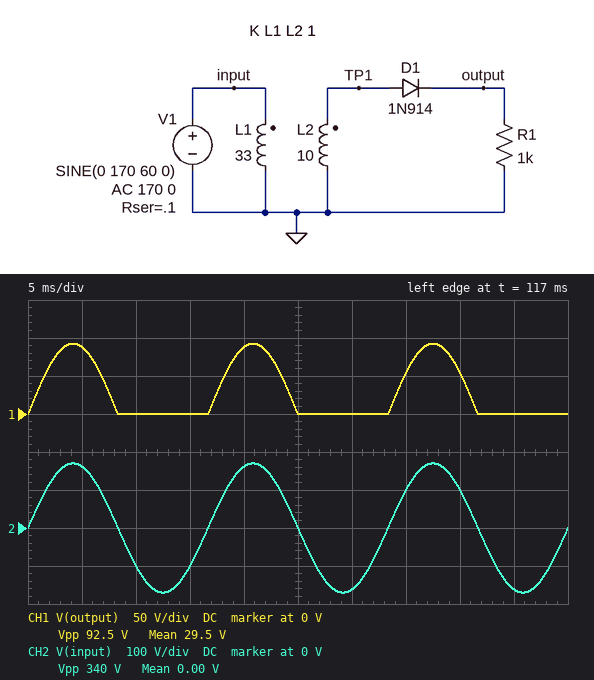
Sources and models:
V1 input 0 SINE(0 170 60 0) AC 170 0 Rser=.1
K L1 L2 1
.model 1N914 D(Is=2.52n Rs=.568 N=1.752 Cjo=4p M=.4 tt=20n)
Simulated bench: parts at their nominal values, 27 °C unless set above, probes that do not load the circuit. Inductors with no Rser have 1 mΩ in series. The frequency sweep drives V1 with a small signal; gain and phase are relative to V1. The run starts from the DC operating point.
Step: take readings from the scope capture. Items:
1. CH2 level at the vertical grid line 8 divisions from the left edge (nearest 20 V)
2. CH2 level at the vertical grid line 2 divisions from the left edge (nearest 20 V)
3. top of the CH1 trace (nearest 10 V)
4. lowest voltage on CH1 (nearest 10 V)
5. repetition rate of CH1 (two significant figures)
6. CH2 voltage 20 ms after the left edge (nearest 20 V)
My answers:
100 V
-100 V
90 V
0 V
60 Hz
160 V
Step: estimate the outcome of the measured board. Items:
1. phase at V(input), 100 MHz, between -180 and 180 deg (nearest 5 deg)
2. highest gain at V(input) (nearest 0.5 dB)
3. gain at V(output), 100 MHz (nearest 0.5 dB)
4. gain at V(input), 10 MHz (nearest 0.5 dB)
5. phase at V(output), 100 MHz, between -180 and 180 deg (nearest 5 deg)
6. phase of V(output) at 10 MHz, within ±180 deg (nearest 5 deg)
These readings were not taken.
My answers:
0 deg
0 dB
-6.0 dB
0 dB
20 deg
75 deg
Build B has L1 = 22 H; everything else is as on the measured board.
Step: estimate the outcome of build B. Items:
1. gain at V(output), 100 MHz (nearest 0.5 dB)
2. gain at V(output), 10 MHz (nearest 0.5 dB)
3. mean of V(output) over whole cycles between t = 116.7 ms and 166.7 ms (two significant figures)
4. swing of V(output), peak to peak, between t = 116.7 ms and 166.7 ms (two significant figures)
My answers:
-4.0 dB
-15.5 dB
36 V
110 V
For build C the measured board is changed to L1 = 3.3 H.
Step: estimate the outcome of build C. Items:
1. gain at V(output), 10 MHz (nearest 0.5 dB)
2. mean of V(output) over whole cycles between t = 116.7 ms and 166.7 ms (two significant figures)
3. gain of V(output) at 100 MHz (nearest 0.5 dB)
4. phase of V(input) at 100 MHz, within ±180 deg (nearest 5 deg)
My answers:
-7.5 dB
94 V
4.0 dB
0 deg
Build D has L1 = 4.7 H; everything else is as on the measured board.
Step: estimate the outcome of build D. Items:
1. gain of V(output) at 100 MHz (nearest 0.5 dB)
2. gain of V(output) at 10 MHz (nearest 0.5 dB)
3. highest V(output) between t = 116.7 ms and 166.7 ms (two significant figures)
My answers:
2.5 dB
-9.0 dB
250 V
